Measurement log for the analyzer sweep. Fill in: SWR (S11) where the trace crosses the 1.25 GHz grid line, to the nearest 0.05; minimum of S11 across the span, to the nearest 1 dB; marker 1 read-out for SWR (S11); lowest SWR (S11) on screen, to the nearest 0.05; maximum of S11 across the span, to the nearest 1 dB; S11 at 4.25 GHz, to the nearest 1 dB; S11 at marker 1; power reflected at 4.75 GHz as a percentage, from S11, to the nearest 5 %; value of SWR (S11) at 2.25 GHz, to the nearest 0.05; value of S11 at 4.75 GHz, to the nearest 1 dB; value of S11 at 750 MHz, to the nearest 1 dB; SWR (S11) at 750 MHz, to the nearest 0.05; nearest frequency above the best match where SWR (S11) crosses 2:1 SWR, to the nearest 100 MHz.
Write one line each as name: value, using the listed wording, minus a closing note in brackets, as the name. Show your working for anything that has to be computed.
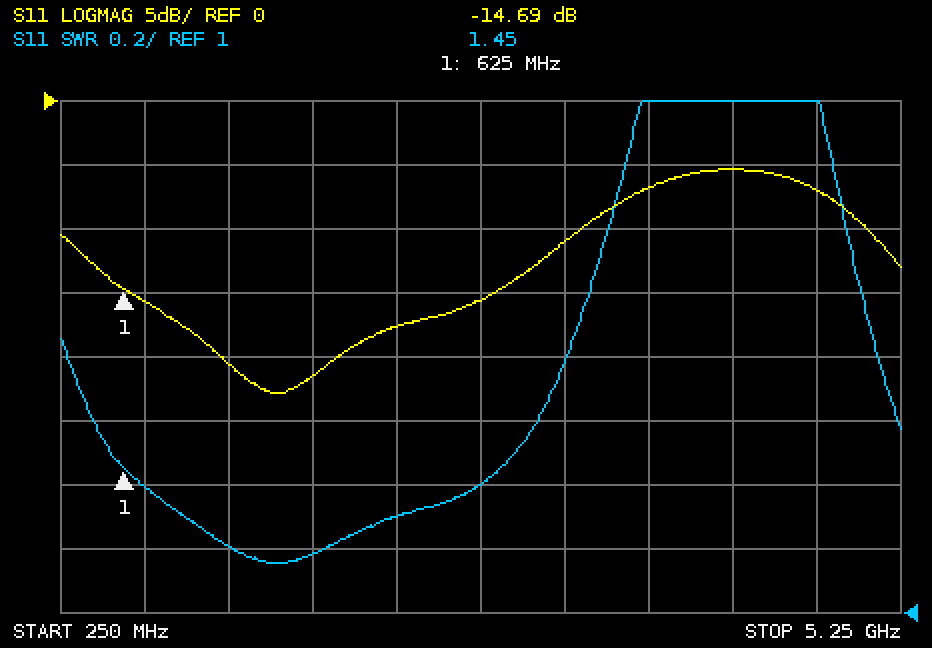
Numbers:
SWR (S11) where the trace crosses the 1.25 GHz grid line, to the nearest 0.05: 1.20
minimum of S11 across the span, to the nearest 1 dB: -23 dB
marker 1 read-out for SWR: 1.45
lowest SWR (S11) on screen, to the nearest 0.05: 1.15
maximum of S11 across the span, to the nearest 1 dB: -5 dB
S11 at 4.25 GHz, to the nearest 1 dB: -5 dB
S11 at marker 1: -14.69 dB
power reflected at 4.75 GHz as a percentage, from S11, to the nearest 5 %: 10^(-7/10) ≈ 20 %
value of SWR (S11) at 2.25 GHz, to the nearest 0.05: 1.30
value of S11 at 4.75 GHz, to the nearest 1 dB: -7 dB
value of S11 at 750 MHz, to the nearest 1 dB: -16 dB
SWR (S11) at 750 MHz, to the nearest 0.05: 1.40
nearest frequency above the best match where SWR (S11) crosses 2:1 SWR, to the nearest 100 MHz: 3.4 GHz
